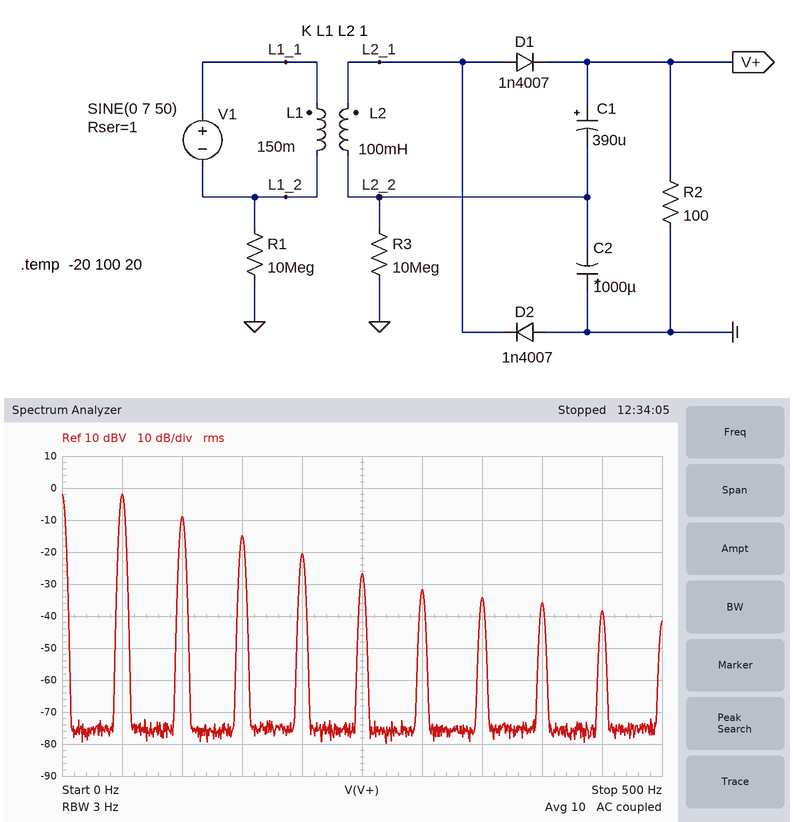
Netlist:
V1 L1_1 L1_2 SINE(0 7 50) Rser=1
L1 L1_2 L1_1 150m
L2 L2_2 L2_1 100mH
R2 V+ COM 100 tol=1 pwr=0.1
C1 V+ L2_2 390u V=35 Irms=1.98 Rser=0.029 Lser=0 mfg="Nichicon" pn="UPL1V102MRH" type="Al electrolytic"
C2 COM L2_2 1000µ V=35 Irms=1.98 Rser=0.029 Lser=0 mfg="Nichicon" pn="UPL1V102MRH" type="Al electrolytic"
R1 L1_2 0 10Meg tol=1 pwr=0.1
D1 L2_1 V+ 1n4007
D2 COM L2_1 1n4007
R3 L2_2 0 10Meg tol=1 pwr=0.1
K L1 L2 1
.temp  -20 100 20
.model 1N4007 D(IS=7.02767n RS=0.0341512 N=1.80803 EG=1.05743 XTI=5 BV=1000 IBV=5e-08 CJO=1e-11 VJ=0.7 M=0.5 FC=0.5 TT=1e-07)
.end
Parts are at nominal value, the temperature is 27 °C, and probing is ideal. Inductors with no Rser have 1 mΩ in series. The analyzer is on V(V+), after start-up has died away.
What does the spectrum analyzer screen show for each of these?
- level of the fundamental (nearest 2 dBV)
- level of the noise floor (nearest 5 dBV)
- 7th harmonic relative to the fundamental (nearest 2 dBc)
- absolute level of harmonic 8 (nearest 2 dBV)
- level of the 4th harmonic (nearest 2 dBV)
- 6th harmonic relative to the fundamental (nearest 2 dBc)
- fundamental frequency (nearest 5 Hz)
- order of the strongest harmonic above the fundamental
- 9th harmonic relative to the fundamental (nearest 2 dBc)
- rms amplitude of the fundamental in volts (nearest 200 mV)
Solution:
-2 dBV
-75 dBV
-32 dBc
-36 dBV
-20 dBV
-30 dBc
50 Hz
2
-36 dBc
800 mV
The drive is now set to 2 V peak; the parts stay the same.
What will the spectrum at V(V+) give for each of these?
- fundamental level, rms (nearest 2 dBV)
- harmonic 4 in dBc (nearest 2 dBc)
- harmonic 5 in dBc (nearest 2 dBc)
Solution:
-16 dBV
-18 dBc
-22 dBc
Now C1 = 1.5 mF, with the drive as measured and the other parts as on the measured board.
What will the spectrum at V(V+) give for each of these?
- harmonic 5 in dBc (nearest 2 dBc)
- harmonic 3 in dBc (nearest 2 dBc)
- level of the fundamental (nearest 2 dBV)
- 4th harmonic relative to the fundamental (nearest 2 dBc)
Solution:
-20 dBc
-12 dBc
-12 dBV
-16 dBc
